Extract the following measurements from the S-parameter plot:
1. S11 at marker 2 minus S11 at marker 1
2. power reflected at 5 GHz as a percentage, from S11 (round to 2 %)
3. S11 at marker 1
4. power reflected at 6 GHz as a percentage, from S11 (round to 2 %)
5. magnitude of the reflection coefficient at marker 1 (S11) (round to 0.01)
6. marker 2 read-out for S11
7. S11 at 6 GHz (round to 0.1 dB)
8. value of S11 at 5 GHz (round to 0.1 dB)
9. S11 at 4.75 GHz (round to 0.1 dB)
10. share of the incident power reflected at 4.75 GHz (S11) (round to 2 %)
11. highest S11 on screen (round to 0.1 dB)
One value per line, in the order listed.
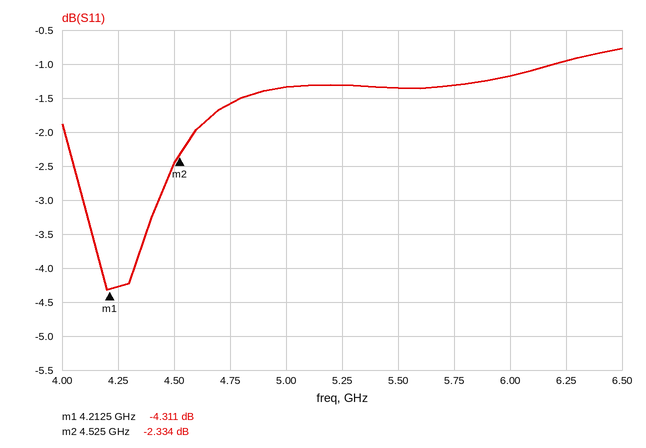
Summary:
1.977 dB
74 %
-4.311 dB
76 %
0.61
-2.334 dB
-1.2 dB
-1.3 dB
-1.6 dB
70 %
-0.8 dB
